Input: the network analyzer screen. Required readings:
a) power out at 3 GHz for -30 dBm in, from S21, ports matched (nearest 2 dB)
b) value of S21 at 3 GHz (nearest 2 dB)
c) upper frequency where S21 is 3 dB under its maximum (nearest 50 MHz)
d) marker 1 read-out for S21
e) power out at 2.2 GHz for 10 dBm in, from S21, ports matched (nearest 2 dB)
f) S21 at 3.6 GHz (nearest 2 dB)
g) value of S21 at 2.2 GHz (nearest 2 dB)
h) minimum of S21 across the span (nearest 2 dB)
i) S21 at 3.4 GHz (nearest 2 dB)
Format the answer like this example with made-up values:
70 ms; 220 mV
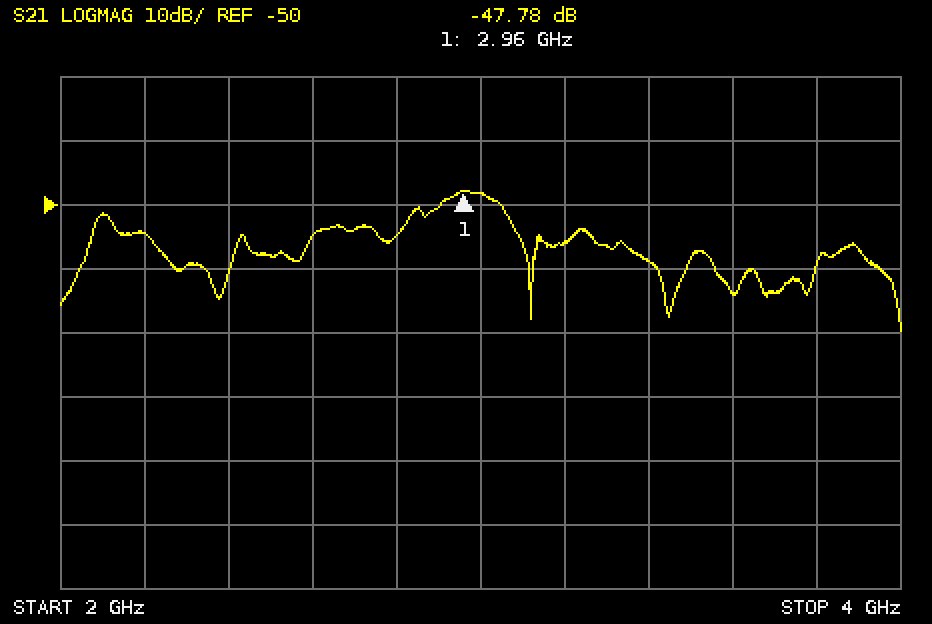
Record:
-78 dBm; -48 dB; 3.05 GHz; -47.78 dB; -44 dBm; -64 dB; -54 dB; -70 dB; -58 dB
